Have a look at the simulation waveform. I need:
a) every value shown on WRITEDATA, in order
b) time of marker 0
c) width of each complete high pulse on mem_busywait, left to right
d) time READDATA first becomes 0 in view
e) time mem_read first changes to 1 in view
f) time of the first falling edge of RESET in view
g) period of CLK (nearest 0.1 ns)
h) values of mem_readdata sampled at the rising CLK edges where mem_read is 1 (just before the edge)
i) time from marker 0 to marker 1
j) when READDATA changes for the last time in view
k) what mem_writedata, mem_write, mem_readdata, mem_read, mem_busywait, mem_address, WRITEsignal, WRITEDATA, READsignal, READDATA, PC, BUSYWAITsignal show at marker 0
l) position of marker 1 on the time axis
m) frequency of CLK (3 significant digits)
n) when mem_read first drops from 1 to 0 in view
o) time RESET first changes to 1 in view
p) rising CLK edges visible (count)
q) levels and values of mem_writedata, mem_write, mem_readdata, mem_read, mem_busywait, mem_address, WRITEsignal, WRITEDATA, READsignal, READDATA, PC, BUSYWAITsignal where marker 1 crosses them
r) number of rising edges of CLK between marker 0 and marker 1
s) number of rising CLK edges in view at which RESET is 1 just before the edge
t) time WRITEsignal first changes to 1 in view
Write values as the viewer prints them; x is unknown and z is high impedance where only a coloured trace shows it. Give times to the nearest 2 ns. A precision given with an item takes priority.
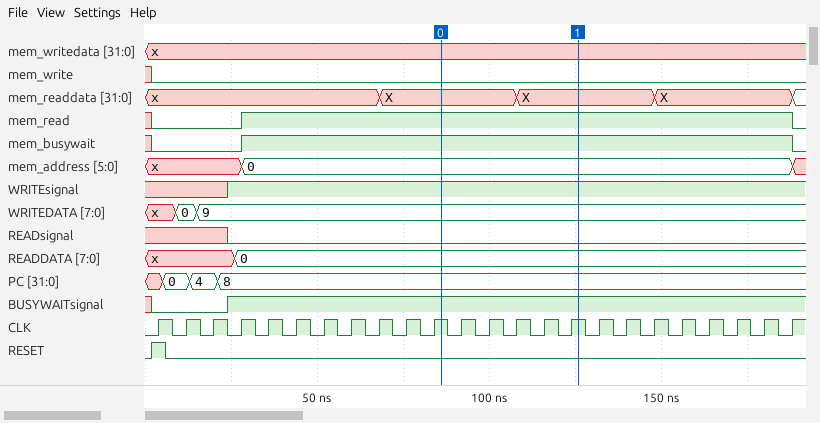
x, 0, 9
86 ns
160 ns
26 ns
28 ns
6 ns
8 ns
x, x, x, x, x, X, X, X, X, X, X, X, X, X, X, X, X, X, X, X
40 ns
26 ns
mem_writedata=x, mem_write=0, mem_readdata=X, mem_read=1, mem_busywait=1, mem_address=0, WRITEsignal=1, WRITEDATA=9, READsignal=0, READDATA=0, PC=8, BUSYWAITsignal=1
126 ns
125 MHz
188 ns
2 ns
24
mem_writedata=x, mem_write=0, mem_readdata=X, mem_read=1, mem_busywait=1, mem_address=0, WRITEsignal=1, WRITEDATA=9, READsignal=0, READDATA=0, PC=8, BUSYWAITsignal=1
5
1
24 ns
